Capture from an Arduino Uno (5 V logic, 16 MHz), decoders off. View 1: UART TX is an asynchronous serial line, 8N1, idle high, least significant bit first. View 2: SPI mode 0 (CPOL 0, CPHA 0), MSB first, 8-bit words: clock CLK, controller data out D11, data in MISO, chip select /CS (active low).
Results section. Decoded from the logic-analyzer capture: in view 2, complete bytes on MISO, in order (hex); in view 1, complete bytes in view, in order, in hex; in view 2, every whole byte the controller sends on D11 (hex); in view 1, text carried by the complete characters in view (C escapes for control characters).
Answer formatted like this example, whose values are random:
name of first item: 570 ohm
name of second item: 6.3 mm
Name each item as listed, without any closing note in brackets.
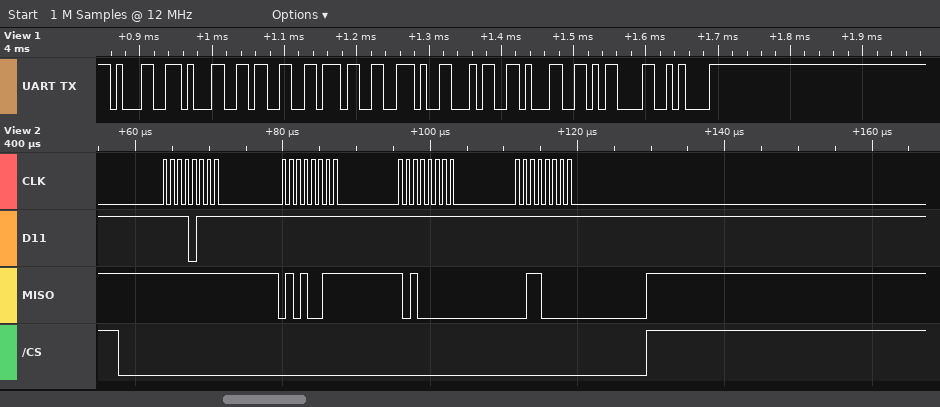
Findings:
in view 2, complete bytes on MISO, in order: FF 53 A0 30
in view 1, complete bytes in view, in order, in hex: 31 31 33 37 2E 34 31 0D 0A
in view 2, every whole byte the controller sends on D11: F7 FF FF FF
in view 1, text carried by the complete characters in view: "1137.41\r\n"
